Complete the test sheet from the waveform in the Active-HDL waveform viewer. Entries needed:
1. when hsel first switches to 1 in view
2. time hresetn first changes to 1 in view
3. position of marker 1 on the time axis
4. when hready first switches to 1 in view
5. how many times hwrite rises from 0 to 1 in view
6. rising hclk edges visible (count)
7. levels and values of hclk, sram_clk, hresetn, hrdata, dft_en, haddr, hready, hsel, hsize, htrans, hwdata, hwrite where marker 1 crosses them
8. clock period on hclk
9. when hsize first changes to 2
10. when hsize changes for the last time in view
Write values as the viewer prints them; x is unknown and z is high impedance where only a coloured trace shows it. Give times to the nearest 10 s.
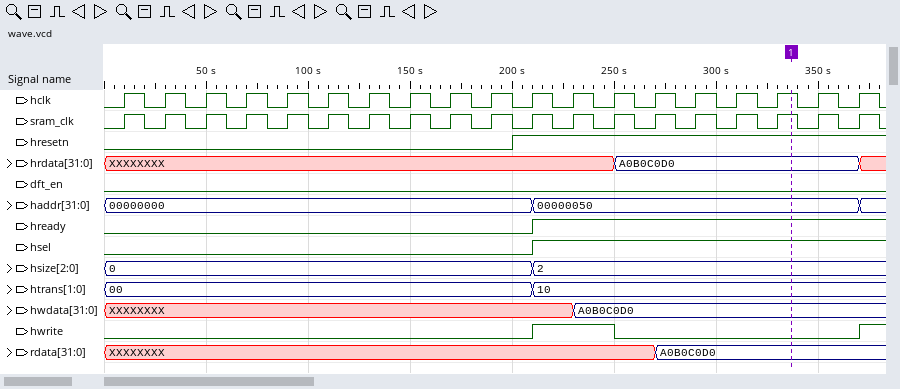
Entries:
210 s
200 s
340 s
210 s
2
19
hclk=1, sram_clk=1, hresetn=1, hrdata=A0B0C0D0, dft_en=0, haddr=00000050, hready=1, hsel=1, hsize=2, htrans=10, hwdata=A0B0C0D0, hwrite=0
20 s
210 s
210 s
